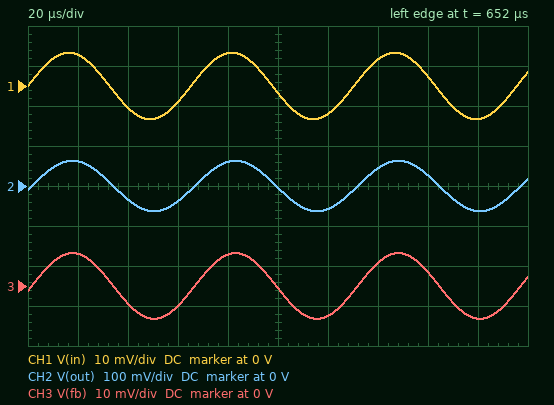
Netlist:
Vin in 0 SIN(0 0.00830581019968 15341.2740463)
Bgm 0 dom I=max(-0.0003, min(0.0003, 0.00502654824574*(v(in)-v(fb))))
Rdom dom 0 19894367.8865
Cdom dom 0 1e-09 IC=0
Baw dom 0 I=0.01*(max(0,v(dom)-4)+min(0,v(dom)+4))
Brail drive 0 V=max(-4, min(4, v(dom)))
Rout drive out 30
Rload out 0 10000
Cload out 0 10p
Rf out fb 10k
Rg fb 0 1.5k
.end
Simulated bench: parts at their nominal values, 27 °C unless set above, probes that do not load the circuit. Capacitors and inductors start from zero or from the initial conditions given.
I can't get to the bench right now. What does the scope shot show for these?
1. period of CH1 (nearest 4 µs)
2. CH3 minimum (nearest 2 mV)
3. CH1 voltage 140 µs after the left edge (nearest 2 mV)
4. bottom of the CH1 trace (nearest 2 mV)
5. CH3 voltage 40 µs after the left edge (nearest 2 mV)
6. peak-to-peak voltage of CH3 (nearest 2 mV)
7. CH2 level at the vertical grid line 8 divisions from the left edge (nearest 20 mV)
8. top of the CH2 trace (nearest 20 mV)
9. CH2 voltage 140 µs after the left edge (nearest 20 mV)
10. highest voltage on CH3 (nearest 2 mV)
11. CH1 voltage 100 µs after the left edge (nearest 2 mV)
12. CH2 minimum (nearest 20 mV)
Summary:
64 µs
-8 mV
6 mV
-8 mV
-4 mV
16 mV
20 mV
60 mV
40 mV
8 mV
-2 mV
-60 mV
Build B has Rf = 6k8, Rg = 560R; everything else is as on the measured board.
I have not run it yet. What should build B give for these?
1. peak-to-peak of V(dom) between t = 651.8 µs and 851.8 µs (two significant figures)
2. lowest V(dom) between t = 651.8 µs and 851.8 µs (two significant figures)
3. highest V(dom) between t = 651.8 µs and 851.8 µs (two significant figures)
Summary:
210 mV
-110 mV
110 mV
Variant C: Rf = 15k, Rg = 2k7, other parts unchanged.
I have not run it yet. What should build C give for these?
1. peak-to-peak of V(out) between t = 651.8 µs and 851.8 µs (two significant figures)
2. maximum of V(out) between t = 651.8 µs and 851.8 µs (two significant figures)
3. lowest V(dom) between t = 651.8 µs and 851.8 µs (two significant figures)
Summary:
110 mV
54 mV
-54 mV
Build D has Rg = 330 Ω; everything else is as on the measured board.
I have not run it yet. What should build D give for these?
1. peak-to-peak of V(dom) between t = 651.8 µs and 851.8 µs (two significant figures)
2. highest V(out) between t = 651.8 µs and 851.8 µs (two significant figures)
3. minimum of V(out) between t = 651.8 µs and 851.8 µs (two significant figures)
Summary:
450 mV
220 mV
-220 mV
